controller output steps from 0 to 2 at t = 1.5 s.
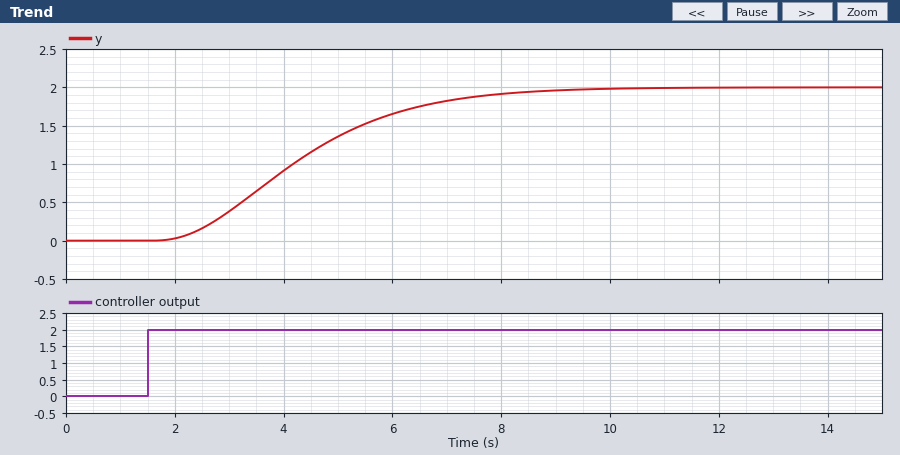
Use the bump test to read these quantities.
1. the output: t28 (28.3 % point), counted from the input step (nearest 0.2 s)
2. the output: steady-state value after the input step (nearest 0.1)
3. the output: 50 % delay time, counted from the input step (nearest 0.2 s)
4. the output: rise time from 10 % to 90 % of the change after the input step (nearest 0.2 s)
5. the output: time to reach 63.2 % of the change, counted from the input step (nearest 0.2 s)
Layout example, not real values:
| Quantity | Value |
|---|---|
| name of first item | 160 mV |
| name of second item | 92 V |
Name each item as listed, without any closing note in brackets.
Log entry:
| Quantity | Value |
|---|---|
| the output: t28 (28.3 % point), counted from the input step | 1.8 s |
| the output: steady-state value after the input step | 2.0 |
| the output: 50 % delay time, counted from the input step | 2.6 s |
| the output: rise time from 10 % to 90 % of the change after the input step | 4.2 s |
| the output: time to reach 63.2 % of the change, counted from the input step | 3.2 s |
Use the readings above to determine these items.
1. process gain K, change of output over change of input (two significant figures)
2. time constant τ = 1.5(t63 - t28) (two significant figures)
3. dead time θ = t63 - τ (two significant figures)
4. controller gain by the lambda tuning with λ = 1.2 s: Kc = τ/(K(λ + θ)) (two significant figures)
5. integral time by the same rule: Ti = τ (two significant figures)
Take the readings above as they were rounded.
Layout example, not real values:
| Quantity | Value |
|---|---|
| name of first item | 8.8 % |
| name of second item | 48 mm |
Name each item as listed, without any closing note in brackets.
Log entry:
| Quantity | Value |
|---|---|
| process gain K, change of output over change of input | 1.0 |
| time constant τ = 1.5(t63 - t28) | 2.1 s |
| dead time θ = t63 - τ | 1.1 s |
| controller gain by the lambda tuning with λ = 1.2 s: Kc = τ/(K(λ + θ)) | 0.91 |
| integral time by the same rule: Ti = τ | 2.1 s |
